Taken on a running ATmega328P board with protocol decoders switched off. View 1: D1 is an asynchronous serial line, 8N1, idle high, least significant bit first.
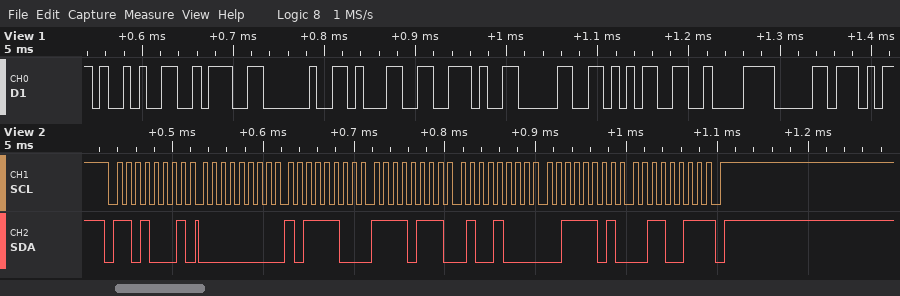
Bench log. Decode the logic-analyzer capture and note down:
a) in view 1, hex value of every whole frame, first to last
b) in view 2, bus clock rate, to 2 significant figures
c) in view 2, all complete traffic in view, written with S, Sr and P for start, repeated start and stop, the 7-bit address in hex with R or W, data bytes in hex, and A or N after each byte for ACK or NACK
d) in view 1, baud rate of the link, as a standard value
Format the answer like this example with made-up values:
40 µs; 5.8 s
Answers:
29 3A 20 31 2E 30 35 C2 B0; 100 kHz; S 68R A 00 A BC A F7 A 48 A 3D A 33 N P; 115200 baud
